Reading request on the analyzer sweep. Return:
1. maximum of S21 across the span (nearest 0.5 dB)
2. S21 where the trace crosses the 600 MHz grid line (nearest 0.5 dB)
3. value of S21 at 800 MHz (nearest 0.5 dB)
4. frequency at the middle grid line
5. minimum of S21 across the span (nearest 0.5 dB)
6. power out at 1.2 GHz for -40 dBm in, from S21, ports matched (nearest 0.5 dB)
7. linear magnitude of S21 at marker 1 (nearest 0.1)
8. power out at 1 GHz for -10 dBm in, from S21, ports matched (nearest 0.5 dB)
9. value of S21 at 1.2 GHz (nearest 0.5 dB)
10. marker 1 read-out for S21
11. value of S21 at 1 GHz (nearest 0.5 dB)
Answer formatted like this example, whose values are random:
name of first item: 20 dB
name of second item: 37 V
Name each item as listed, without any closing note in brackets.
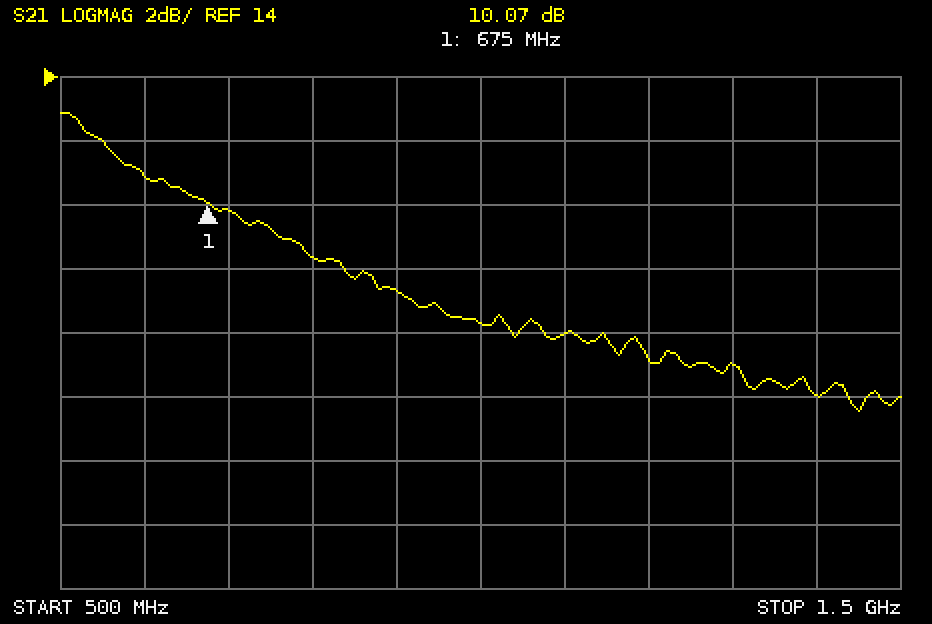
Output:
maximum of S21 across the span: 13.0 dB
S21 where the trace crosses the 600 MHz grid line: 11.0 dB
value of S21 at 800 MHz: 8.5 dB
frequency at the middle grid line: 1 GHz
minimum of S21 across the span: 3.5 dB
power out at 1.2 GHz for -40 dBm in, from S21, ports matched: -35.0 dBm
linear magnitude of S21 at marker 1: 3.2
power out at 1 GHz for -10 dBm in, from S21, ports matched: -3.5 dBm
value of S21 at 1.2 GHz: 5.0 dB
marker 1 read-out for S21: 10.07 dB
value of S21 at 1 GHz: 6.5 dB
